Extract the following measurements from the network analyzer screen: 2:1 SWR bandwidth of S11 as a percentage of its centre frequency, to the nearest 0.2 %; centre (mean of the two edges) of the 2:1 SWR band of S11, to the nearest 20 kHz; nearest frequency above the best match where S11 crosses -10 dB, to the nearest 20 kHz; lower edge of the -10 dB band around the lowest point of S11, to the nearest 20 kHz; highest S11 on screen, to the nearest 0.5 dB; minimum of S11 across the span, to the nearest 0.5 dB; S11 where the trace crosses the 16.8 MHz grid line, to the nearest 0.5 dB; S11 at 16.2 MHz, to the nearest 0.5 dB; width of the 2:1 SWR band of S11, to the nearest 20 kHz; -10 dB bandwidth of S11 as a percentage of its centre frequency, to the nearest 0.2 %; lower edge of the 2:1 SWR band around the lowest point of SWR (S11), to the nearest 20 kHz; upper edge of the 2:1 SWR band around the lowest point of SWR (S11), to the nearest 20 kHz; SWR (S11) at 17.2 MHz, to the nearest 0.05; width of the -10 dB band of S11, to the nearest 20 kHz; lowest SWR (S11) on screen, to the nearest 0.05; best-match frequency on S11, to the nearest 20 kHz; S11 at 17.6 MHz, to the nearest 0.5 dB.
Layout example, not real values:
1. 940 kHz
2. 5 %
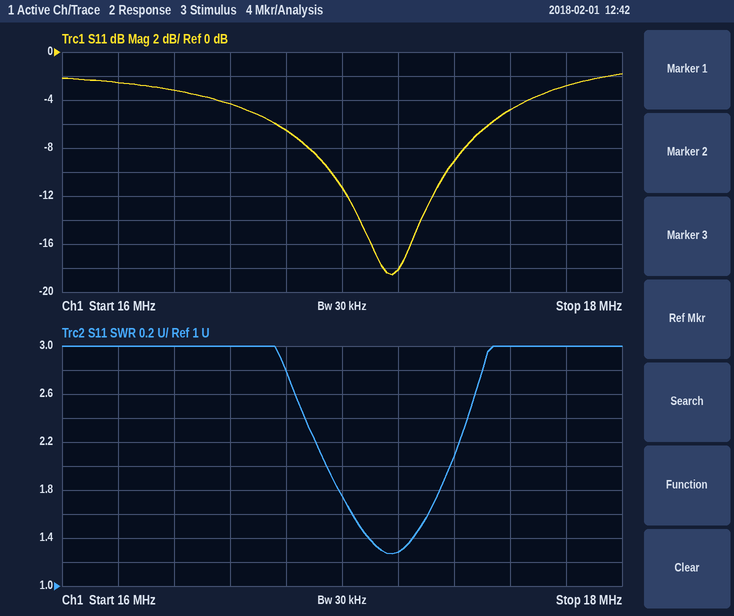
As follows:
1. 2.6 %
2. 17.16 MHz
3. 17.38 MHz
4. 16.96 MHz
5. -2.0 dB
6. -18.5 dB
7. -6.5 dB
8. -2.5 dB
9. 440 kHz
10. 2.4 %
11. 16.94 MHz
12. 17.38 MHz
13. 1.30
14. 420 kHz
15. 1.25
16. 17.18 MHz
17. -5.0 dB
